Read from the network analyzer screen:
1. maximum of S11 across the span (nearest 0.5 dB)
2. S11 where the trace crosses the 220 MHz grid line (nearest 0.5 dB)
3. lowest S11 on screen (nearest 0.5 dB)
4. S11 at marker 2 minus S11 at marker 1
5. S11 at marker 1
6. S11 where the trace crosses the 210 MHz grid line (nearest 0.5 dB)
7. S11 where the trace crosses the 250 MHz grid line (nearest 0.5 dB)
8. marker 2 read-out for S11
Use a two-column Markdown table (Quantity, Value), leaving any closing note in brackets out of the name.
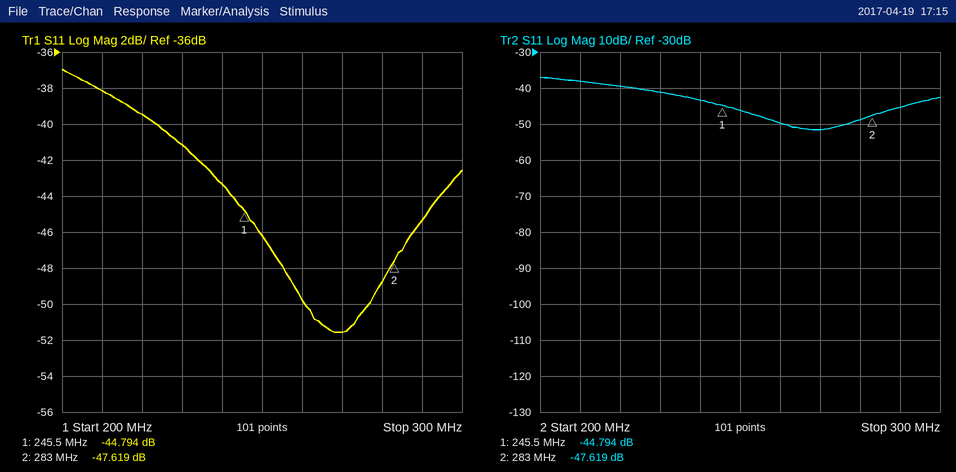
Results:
| Quantity | Value |
|---|---|
| maximum of S11 across the span | -37.0 dB |
| S11 where the trace crosses the 220 MHz grid line | -39.5 dB |
| lowest S11 on screen | -51.5 dB |
| S11 at marker 2 minus S11 at marker 1 | -2.825 dB |
| S11 at marker 1 | -44.794 dB |
| S11 where the trace crosses the 210 MHz grid line | -38.0 dB |
| S11 where the trace crosses the 250 MHz grid line | -46.0 dB |
| marker 2 read-out for S11 | -47.619 dB |
